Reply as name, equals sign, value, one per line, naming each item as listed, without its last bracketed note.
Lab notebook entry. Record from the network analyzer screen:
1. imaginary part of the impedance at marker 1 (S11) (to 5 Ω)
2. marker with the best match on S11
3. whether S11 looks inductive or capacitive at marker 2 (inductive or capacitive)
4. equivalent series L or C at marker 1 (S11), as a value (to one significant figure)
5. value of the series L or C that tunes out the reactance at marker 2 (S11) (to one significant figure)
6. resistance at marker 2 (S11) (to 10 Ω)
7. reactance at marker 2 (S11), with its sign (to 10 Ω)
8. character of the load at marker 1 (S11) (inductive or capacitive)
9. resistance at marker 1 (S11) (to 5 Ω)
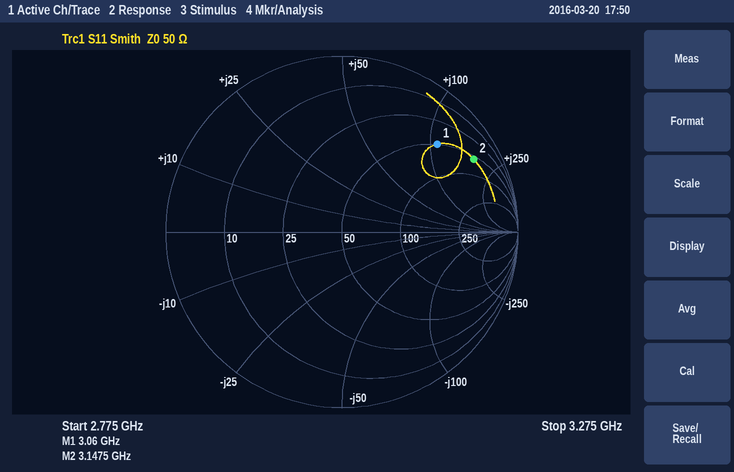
imaginary part of the impedance at marker 1 (S11) = +110 Ω
marker with the best match on S11 = marker 1
whether S11 looks inductive or capacitive at marker 2 = inductive
equivalent series L or C at marker 1 (S11), as a value = 6 nH
value of the series L or C that tunes out the reactance at marker 2 (S11) = 300 fF
resistance at marker 2 (S11) = 60 Ω
reactance at marker 2 (S11), with its sign = +180 Ω
character of the load at marker 1 (S11) = inductive
resistance at marker 1 (S11) = 50 Ω
